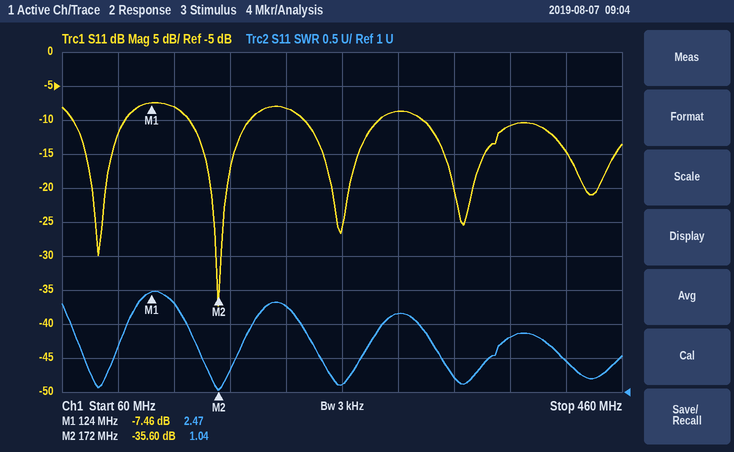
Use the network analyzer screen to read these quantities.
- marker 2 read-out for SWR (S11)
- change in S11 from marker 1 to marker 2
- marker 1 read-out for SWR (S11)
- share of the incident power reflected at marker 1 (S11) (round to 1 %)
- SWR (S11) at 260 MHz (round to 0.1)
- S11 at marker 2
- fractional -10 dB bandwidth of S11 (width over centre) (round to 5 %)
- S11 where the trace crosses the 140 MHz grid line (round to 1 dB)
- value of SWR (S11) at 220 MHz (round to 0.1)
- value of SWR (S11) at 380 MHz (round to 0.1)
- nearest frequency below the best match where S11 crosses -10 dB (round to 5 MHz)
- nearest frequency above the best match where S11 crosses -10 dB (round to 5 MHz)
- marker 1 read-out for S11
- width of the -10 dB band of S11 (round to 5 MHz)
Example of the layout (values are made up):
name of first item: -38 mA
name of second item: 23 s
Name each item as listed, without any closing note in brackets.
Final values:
marker 2 read-out for SWR: 1.04
change in S11 from marker 1 to marker 2: -28.14 dB
marker 1 read-out for SWR: 2.47
share of the incident power reflected at marker 1 (S11): 18 %
SWR (S11) at 260 MHz: 1.1
S11 at marker 2: -35.60 dB
fractional -10 dB bandwidth of S11 (width over centre): 25 %
S11 where the trace crosses the 140 MHz grid line: -8 dB
value of SWR (S11) at 220 MHz: 2.3
value of SWR (S11) at 380 MHz: 1.8
nearest frequency below the best match where S11 crosses -10 dB: 150 MHz
nearest frequency above the best match where S11 crosses -10 dB: 195 MHz
marker 1 read-out for S11: -7.46 dB
width of the -10 dB band of S11: 45 MHz
